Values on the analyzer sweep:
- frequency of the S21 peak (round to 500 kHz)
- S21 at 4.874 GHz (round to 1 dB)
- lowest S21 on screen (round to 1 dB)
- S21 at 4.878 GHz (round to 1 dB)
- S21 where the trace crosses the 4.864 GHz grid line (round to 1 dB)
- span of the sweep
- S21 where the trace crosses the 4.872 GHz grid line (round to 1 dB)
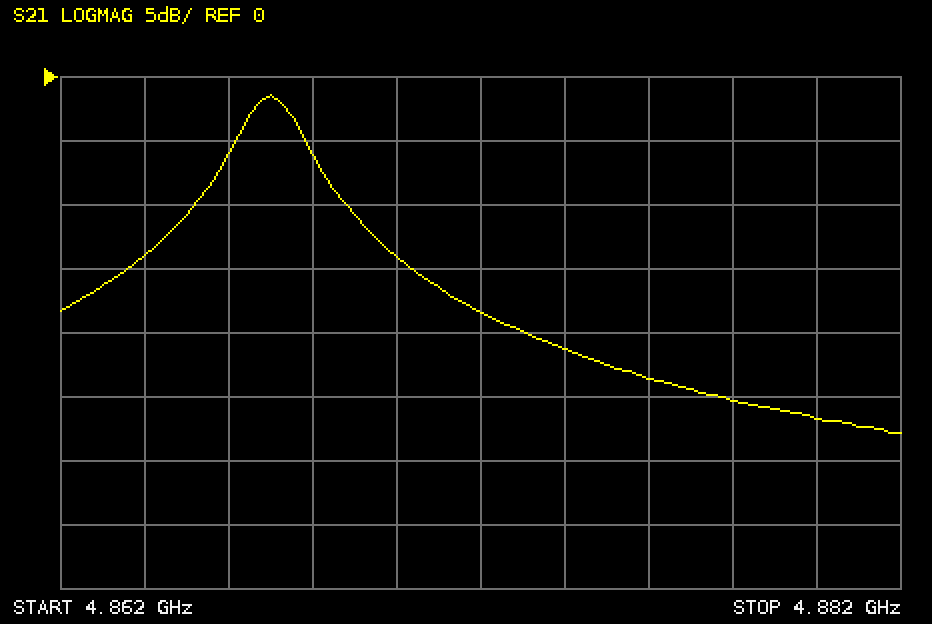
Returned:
4.8670 GHz
-21 dB
-28 dB
-25 dB
-14 dB
20 MHz
-18 dB
